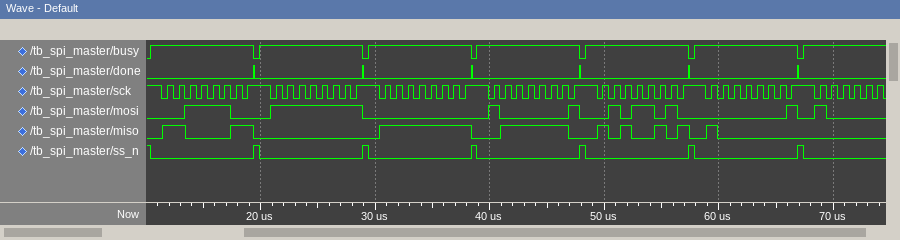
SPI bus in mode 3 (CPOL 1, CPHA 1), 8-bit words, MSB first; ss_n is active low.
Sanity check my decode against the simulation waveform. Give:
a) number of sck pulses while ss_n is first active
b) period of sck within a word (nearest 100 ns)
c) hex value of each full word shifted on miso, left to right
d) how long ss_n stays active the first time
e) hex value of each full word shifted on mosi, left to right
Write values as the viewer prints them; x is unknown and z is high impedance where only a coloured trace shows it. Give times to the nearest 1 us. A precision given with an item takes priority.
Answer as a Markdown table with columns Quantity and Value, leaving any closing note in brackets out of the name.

| Quantity | Value |
|---|---|
| number of sck pulses while ss_n is first active | 8 |
| period of sck within a word | 1000 ns |
| hex value of each full word shifted on miso, left to right | C3, 00, FF, 7E, A5, 80 |
| how long ss_n stays active the first time | 9 us |
| hex value of each full word shifted on mosi, left to right | 3C, FF, 00, 81, 5A, 01 |
